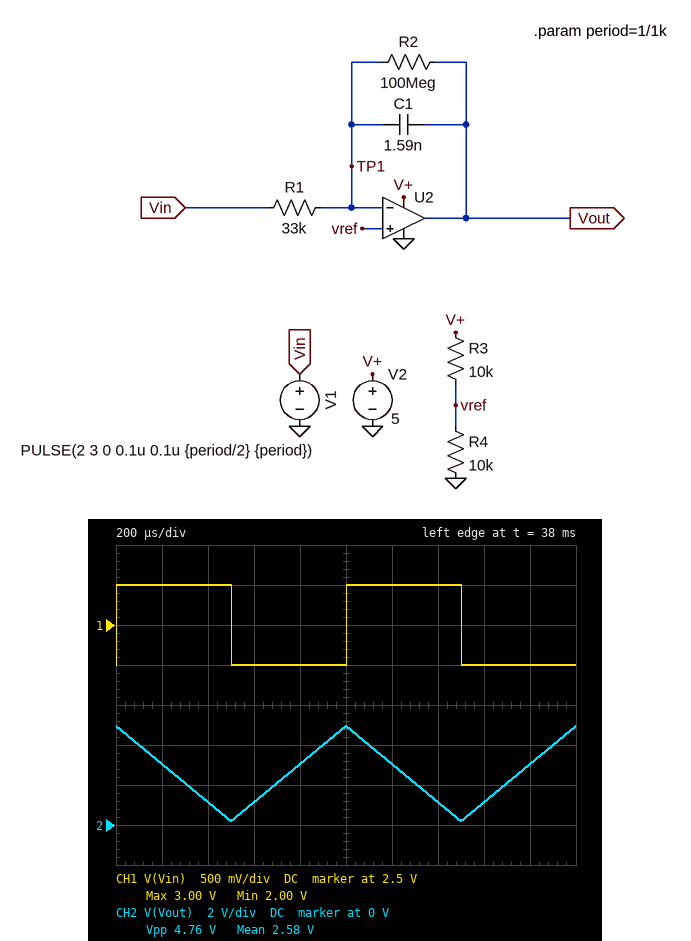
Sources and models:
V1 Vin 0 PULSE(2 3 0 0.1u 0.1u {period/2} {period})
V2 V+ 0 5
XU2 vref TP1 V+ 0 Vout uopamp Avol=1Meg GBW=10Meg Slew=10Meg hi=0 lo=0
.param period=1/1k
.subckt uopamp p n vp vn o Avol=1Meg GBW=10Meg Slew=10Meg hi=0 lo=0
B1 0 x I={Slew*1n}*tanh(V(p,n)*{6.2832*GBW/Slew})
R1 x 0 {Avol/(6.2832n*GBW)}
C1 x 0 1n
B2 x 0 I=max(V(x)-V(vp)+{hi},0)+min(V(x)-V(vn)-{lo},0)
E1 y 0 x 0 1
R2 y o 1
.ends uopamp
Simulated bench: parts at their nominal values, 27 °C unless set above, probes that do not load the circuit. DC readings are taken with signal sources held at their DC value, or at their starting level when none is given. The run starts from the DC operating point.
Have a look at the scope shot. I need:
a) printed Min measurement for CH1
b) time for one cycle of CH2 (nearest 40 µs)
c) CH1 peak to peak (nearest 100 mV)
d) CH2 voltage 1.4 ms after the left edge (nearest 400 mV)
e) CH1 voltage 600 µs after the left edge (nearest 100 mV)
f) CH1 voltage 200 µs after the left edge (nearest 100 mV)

2.00 V
1.00 ms
1.0 V
1.2 V
2.0 V
3.0 V
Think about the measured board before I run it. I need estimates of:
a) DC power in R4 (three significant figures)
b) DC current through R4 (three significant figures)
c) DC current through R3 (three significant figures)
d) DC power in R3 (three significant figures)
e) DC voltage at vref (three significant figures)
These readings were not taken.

625 µW
250 µA
250 µA
625 µW
2.50 V
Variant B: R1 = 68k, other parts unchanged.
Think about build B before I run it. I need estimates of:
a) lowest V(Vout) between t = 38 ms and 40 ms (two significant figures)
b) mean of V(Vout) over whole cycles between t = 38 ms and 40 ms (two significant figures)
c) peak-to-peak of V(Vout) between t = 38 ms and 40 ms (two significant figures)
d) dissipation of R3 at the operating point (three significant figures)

2.4 V
3.6 V
2.3 V
625 µW
